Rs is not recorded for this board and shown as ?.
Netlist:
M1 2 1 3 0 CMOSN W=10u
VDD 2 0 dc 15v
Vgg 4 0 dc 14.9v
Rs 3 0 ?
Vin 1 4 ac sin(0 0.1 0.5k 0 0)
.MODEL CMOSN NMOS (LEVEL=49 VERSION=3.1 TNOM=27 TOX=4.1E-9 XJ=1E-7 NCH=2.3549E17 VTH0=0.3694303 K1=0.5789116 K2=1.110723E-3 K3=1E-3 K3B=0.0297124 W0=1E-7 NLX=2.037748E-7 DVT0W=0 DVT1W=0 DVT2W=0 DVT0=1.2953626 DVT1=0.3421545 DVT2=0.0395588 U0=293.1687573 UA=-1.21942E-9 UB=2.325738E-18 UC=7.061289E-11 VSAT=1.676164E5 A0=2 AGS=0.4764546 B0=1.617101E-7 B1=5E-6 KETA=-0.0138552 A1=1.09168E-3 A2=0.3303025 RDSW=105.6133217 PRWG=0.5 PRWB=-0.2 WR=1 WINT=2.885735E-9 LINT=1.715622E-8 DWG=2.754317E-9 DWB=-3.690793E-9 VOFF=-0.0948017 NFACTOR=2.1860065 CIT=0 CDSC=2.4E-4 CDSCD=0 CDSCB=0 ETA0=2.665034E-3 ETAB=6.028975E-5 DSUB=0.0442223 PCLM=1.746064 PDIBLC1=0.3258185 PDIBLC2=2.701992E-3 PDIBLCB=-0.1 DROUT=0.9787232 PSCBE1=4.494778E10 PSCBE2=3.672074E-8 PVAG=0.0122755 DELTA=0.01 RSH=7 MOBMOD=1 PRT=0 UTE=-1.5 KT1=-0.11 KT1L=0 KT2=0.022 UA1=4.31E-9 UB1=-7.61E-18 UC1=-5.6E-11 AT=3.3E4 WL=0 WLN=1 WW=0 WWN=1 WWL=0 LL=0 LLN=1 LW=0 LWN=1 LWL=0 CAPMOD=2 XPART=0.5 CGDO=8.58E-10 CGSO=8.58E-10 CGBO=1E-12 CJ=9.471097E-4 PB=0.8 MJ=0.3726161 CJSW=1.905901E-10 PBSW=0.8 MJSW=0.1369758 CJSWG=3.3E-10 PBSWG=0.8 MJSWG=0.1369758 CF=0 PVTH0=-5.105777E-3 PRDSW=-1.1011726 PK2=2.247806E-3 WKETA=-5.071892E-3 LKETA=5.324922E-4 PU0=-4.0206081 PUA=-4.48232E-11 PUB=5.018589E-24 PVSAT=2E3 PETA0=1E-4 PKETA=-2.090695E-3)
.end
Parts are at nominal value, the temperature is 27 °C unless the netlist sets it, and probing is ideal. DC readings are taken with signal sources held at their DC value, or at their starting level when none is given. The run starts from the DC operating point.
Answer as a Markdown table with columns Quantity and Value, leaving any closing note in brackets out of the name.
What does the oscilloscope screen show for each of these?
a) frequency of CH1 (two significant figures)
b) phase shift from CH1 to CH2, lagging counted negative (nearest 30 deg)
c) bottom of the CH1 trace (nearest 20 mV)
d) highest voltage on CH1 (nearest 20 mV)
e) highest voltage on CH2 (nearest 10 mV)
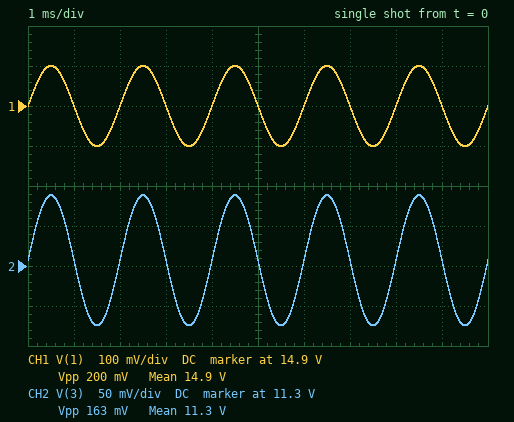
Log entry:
| Quantity | Value |
|---|---|
| frequency of CH1 | 500 Hz |
| phase shift from CH1 to CH2, lagging counted negative | 0 deg |
| bottom of the CH1 trace | 14.80 V |
| highest voltage on CH1 | 15.00 V |
| highest voltage on CH2 | 11.39 V |
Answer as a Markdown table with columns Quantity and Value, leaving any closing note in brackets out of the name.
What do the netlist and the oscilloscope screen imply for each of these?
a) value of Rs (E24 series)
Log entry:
| Quantity | Value |
|---|---|
| value of Rs | 33 kΩ |
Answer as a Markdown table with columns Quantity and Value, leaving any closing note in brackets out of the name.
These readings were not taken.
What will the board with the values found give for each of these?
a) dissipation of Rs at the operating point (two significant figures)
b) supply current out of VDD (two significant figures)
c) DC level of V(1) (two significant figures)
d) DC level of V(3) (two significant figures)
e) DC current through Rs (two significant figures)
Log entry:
| Quantity | Value |
|---|---|
| dissipation of Rs at the operating point | 3.9 mW |
| supply current out of VDD | 340 µA |
| DC level of V(1) | 15 V |
| DC level of V(3) | 11 V |
| DC current through Rs | 340 µA |
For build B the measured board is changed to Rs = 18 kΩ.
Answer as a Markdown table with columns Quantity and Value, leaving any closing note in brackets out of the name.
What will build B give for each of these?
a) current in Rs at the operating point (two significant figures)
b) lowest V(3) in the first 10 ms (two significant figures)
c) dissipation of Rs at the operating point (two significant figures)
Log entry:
| Quantity | Value |
|---|---|
| current in Rs at the operating point | 580 µA |
| lowest V(3) in the first 10 ms | 10 V |
| dissipation of Rs at the operating point | 6.1 mW |
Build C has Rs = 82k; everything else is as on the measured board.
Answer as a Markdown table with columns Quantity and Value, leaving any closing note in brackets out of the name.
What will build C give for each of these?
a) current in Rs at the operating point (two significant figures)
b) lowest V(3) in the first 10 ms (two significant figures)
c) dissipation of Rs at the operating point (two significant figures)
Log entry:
| Quantity | Value |
|---|---|
| current in Rs at the operating point | 150 µA |
| lowest V(3) in the first 10 ms | 12 V |
| dissipation of Rs at the operating point | 1.8 mW |
